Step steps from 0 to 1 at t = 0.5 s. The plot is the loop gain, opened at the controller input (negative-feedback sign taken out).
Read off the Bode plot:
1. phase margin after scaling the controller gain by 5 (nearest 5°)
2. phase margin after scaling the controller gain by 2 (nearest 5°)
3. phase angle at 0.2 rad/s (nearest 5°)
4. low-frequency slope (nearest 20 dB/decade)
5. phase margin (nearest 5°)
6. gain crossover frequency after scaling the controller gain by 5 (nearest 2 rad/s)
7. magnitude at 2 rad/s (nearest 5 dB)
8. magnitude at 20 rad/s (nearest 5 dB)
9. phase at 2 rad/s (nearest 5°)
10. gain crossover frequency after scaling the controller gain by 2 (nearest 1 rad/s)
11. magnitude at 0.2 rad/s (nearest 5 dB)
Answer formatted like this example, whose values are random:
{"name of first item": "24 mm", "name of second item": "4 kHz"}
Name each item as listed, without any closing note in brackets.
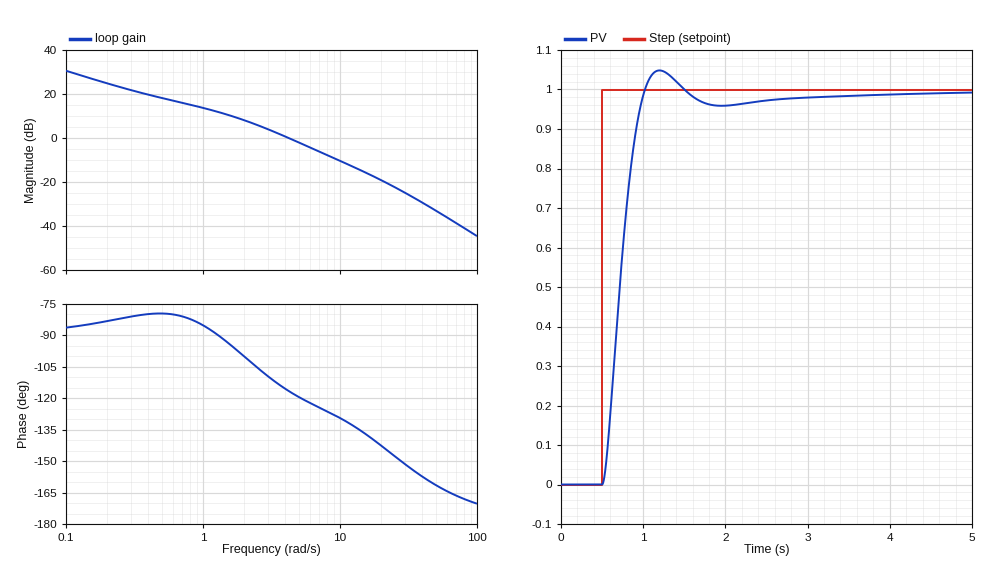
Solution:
{"phase margin after scaling the controller gain by 5": "45°", "phase margin after scaling the controller gain by 2": "55°", "phase angle at 0.2 rad/s": "-85°", "low-frequency slope": "-20 dB/decade", "phase margin": "65°", "gain crossover frequency after scaling the controller gain by 5": "14 rad/s", "magnitude at 2 rad/s": "10 dB", "magnitude at 20 rad/s": "-20 dB", "phase at 2 rad/s": "-100°", "gain crossover frequency after scaling the controller gain by 2": "7 rad/s", "magnitude at 0.2 rad/s": "25 dB"}
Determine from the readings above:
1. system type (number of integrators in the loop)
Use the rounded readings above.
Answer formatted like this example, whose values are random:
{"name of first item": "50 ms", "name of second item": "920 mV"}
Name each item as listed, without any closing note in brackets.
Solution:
{"system type": "1"}
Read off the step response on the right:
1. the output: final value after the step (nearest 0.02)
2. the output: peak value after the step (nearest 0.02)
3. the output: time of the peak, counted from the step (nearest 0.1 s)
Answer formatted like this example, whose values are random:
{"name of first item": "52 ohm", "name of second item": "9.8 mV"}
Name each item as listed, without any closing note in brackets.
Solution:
{"the output: final value after the step": "1.00", "the output: peak value after the step": "1.04", "the output: time of the peak, counted from the step": "0.7 s"}
